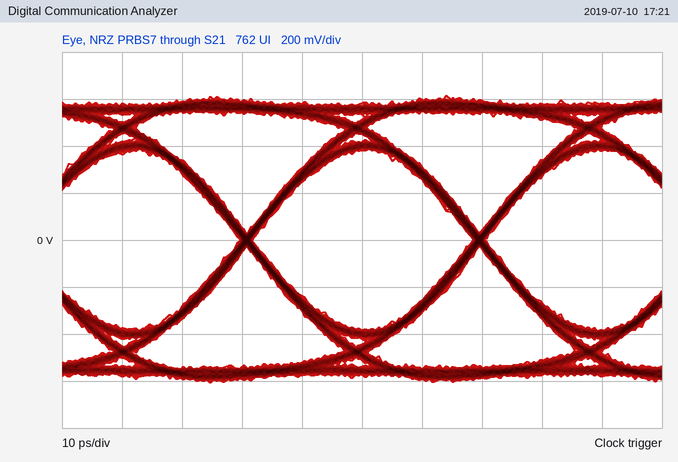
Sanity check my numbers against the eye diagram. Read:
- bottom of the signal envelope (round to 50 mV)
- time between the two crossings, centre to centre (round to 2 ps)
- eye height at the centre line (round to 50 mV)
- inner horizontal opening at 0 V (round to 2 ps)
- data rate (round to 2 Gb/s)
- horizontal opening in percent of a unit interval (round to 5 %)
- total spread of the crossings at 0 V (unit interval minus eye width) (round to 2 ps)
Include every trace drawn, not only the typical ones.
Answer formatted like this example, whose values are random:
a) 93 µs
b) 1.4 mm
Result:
a) -600 mV
b) 38 ps
c) 750 mV
d) 36 ps
e) 26 Gb/s
f) 95 %
g) 2 ps
